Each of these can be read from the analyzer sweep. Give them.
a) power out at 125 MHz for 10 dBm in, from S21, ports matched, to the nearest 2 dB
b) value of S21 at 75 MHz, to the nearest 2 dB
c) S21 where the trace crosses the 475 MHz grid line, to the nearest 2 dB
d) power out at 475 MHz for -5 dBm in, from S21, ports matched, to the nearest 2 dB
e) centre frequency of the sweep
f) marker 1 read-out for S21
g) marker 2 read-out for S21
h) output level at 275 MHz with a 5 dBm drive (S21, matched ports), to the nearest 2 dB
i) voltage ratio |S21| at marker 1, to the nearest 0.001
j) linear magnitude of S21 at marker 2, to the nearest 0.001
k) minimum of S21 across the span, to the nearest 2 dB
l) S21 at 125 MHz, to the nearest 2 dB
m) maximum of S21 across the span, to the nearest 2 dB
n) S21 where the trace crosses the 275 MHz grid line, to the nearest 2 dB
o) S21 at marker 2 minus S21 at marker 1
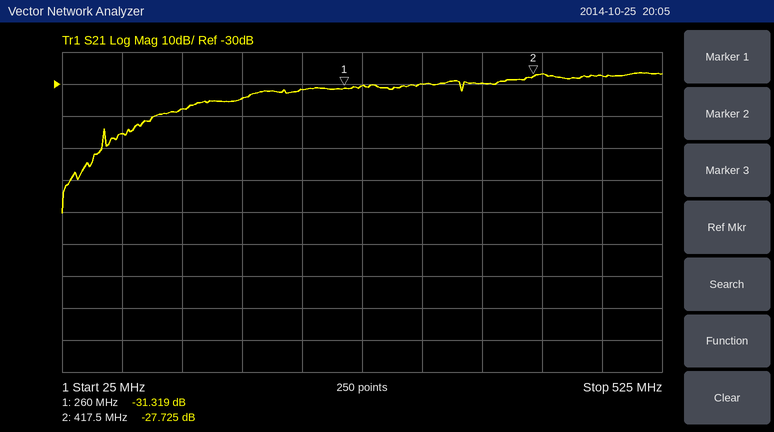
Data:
-28 dBm
-46 dB
-28 dB
-32 dBm
275 MHz
-31.319 dB
-27.725 dB
-26 dBm
0.027
0.041
-70 dB
-38 dB
-26 dB
-30 dB
3.594 dB
